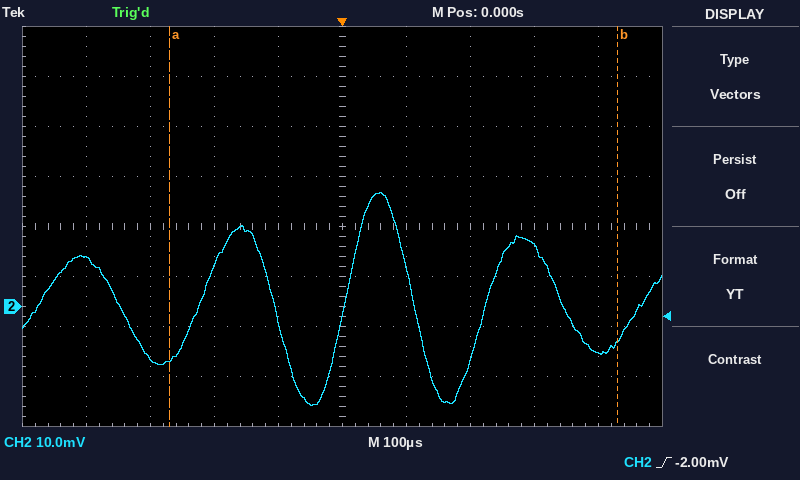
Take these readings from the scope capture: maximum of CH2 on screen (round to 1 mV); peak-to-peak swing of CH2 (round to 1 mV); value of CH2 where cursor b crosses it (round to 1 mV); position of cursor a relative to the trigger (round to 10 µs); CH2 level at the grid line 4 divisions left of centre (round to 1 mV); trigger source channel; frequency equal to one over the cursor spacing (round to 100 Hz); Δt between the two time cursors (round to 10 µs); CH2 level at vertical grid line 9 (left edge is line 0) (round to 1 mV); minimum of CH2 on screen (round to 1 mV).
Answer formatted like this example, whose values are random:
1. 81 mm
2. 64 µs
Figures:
1. 23 mV
2. 43 mV
3. -7 mV
4. -270 µs
5. 10 mV
6. CH2
7. 1.4 kHz
8. 700 µs
9. -9 mV
10. -20 mV
